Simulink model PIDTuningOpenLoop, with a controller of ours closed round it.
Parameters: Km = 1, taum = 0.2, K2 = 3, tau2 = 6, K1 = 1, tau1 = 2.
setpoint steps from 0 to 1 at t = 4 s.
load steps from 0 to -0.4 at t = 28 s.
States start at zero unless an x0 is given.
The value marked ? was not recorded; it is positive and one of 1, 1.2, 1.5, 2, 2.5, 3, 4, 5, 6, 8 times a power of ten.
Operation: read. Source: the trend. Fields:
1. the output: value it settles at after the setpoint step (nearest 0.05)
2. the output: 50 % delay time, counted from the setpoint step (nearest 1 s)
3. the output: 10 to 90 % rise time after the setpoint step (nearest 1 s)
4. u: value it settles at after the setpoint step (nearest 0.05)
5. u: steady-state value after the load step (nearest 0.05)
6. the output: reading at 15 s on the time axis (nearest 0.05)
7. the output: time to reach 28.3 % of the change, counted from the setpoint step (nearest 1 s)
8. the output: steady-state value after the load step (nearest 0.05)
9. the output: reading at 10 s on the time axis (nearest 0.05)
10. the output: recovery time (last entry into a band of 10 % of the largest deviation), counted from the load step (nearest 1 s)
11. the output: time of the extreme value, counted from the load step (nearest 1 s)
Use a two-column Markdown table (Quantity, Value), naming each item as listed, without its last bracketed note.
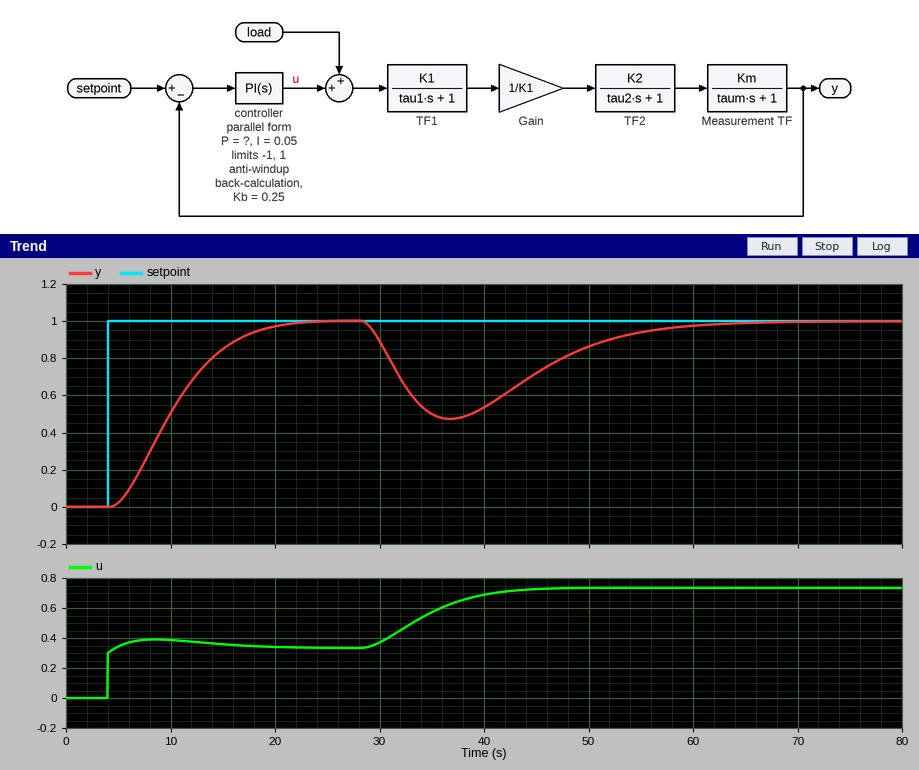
| Quantity | Value |
|---|---|
| the output: value it settles at after the setpoint step | 1.00 |
| the output: 50 % delay time, counted from the setpoint step | 6 s |
| the output: 10 to 90 % rise time after the setpoint step | 10 s |
| u: value it settles at after the setpoint step | 0.35 |
| u: steady-state value after the load step | 0.75 |
| the output: reading at 15 s on the time axis | 0.85 |
| the output: time to reach 28.3 % of the change, counted from the setpoint step | 4 s |
| the output: steady-state value after the load step | 1.00 |
| the output: reading at 10 s on the time axis | 0.50 |
| the output: recovery time (last entry into a band of 10 % of the largest deviation), counted from the load step | 28 s |
| the output: time of the extreme value, counted from the load step | 9 s |
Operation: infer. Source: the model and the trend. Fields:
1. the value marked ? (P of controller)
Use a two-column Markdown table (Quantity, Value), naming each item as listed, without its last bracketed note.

| Quantity | Value |
|---|---|
| the value marked ? | 0.3 |
